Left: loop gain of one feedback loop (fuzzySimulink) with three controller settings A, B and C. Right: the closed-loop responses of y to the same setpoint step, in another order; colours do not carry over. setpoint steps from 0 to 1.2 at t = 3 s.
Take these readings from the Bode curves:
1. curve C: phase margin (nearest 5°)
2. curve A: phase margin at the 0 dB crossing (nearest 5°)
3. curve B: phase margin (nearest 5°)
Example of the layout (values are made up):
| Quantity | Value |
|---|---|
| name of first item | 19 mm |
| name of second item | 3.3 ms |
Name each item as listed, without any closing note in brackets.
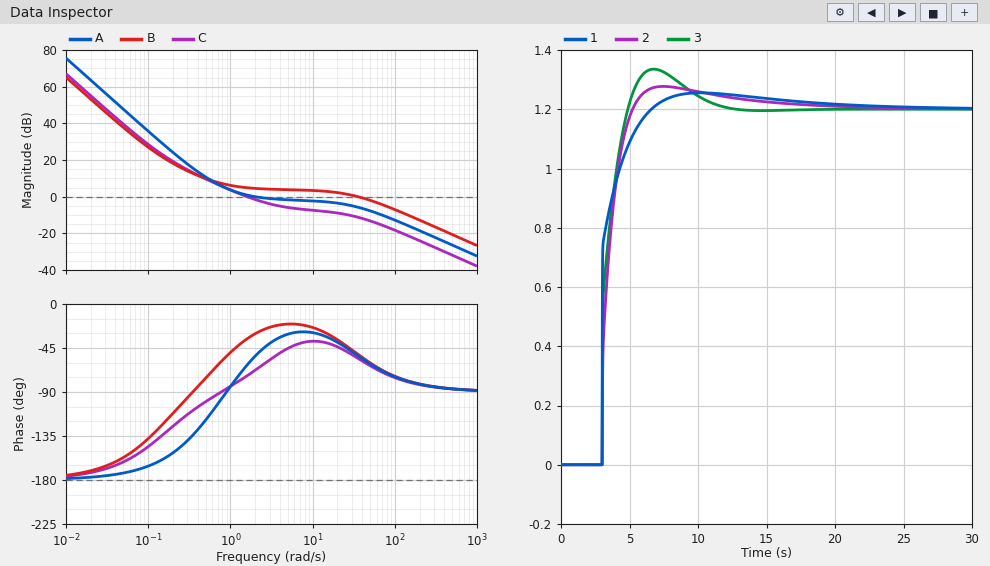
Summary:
| Quantity | Value |
|---|---|
| curve C: phase margin | 105° |
| curve A: phase margin at the 0 dB crossing | 125° |
| curve B: phase margin | 130° |
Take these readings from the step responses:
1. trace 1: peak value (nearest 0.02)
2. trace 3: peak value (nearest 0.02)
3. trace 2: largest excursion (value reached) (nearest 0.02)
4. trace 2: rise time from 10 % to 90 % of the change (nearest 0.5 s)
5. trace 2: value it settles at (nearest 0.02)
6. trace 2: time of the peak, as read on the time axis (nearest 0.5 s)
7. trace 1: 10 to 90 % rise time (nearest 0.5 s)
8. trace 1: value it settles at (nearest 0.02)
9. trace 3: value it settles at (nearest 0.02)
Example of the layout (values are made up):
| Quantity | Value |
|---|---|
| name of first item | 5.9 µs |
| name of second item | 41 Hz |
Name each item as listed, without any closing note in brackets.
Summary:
| Quantity | Value |
|---|---|
| trace 1: peak value | 1.26 |
| trace 3: peak value | 1.34 |
| trace 2: largest excursion (value reached) | 1.28 |
| trace 2: rise time from 10 % to 90 % of the change | 1.5 s |
| trace 2: value it settles at | 1.20 |
| trace 2: time of the peak, as read on the time axis | 7.5 s |
| trace 1: 10 to 90 % rise time | 2.0 s |
| trace 1: value it settles at | 1.20 |
| trace 3: value it settles at | 1.20 |
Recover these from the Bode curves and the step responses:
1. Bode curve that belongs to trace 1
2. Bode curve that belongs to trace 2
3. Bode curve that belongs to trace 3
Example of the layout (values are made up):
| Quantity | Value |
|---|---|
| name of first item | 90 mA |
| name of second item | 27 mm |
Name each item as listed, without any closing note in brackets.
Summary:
| Quantity | Value |
|---|---|
| Bode curve that belongs to trace 1 | B |
| Bode curve that belongs to trace 2 | C |
| Bode curve that belongs to trace 3 | A |
